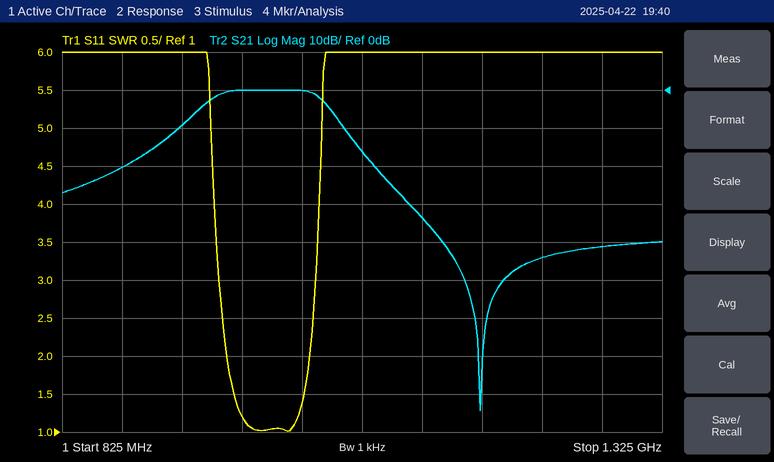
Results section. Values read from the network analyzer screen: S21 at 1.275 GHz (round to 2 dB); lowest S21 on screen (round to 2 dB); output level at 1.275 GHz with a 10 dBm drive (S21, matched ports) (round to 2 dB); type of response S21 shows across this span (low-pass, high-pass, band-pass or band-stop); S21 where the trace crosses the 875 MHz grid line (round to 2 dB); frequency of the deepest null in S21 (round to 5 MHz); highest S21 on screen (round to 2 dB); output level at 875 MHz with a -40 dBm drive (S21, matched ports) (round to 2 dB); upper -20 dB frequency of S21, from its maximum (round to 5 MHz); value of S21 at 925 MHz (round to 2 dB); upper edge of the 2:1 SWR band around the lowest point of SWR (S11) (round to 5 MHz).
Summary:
-42 dB
-84 dB
-32 dBm
band-pass
-20 dB
1.175 GHz
0 dB
-60 dBm
1.085 GHz
-10 dB
1.030 GHz
